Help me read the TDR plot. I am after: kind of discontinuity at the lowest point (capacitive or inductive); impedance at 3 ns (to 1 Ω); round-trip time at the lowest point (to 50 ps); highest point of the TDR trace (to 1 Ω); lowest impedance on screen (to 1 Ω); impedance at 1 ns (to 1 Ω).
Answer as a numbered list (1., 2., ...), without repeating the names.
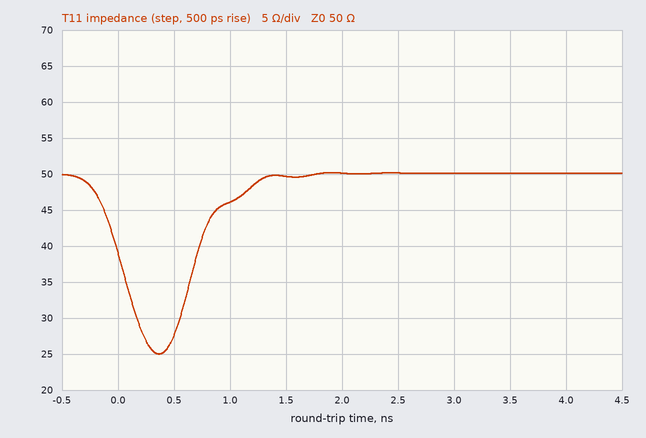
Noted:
1. capacitive
2. 50 Ω
3. 350 ps
4. 50 Ω
5. 25 Ω
6. 46 Ω
